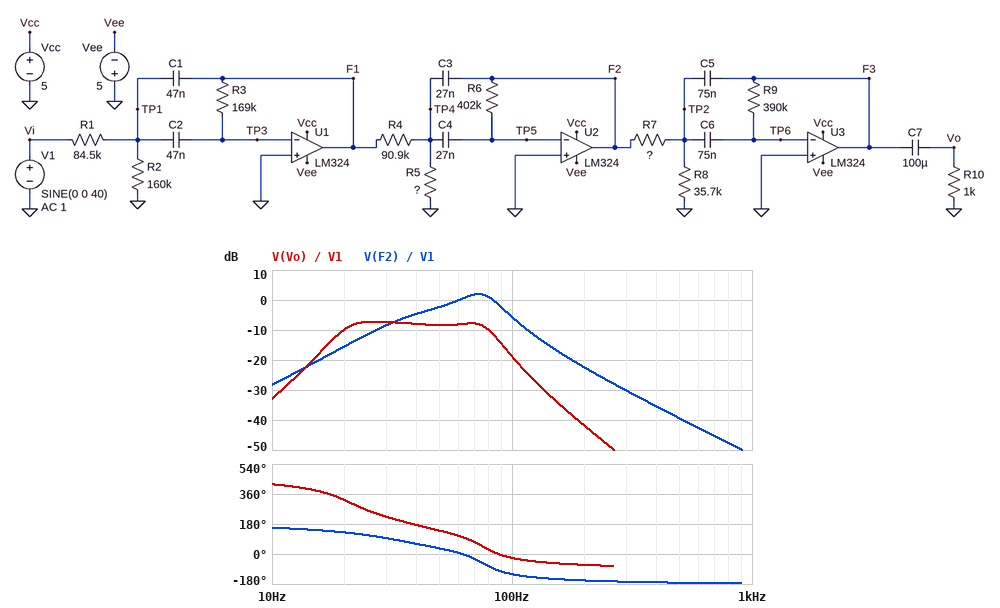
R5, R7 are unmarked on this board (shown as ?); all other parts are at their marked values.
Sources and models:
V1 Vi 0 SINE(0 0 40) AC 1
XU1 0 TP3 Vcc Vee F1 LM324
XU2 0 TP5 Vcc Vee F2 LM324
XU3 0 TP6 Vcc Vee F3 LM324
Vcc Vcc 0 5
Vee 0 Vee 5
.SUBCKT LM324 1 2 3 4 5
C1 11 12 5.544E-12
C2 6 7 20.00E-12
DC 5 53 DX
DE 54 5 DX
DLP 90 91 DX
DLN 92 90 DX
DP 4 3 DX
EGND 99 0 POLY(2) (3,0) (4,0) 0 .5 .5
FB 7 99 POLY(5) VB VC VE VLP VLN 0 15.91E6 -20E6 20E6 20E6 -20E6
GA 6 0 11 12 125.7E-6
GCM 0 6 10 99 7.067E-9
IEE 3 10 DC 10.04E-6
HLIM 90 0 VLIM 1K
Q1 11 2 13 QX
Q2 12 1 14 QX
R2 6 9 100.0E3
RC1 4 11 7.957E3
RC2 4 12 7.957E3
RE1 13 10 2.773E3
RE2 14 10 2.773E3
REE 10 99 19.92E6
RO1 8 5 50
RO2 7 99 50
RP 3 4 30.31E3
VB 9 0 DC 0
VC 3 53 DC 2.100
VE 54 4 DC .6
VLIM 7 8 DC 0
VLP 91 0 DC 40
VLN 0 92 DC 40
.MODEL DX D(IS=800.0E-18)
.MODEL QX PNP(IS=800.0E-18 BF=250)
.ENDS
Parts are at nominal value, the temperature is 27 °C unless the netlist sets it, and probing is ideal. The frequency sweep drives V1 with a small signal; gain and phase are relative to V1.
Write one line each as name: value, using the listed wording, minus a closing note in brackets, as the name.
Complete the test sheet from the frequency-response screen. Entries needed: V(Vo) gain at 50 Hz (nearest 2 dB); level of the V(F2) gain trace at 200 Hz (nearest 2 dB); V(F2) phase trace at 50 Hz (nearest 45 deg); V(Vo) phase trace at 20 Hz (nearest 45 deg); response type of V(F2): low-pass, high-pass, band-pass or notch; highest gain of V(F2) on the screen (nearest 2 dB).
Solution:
V(Vo) gain at 50 Hz: -8 dB
level of the V(F2) gain trace at 200 Hz: -22 dB
V(F2) phase trace at 50 Hz: 45 deg
V(Vo) phase trace at 20 Hz: 315 deg
response type of V(F2): low-pass, high-pass, band-pass or notch: band-pass
highest gain of V(F2) on the screen: 2 dB
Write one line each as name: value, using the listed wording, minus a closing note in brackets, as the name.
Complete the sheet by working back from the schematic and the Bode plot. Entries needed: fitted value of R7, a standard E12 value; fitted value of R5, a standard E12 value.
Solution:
fitted value of R7, a standard E12 value: 100 kΩ
fitted value of R5, a standard E12 value: 18 kΩ
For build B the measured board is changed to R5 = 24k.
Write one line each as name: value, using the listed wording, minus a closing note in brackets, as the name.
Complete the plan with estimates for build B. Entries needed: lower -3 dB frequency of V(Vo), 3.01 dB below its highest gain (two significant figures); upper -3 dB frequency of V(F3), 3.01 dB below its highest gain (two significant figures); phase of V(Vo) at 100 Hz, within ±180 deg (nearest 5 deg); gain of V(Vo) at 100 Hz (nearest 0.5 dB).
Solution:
lower -3 dB frequency of V(Vo), 3.01 dB below its highest gain: 20 Hz
upper -3 dB frequency of V(F3), 3.01 dB below its highest gain: 72 Hz
phase of V(Vo) at 100 Hz, within ±180 deg: -30 deg
gain of V(Vo) at 100 Hz: -20.5 dB
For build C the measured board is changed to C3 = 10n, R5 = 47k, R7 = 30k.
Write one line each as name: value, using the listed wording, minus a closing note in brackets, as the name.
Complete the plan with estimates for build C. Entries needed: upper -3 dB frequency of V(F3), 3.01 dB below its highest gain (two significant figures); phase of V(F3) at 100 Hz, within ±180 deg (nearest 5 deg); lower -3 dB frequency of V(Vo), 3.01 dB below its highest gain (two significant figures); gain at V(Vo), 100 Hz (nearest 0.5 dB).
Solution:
upper -3 dB frequency of V(F3), 3.01 dB below its highest gain: 41 Hz
phase of V(F3) at 100 Hz, within ±180 deg: 5 deg
lower -3 dB frequency of V(Vo), 3.01 dB below its highest gain: 24 Hz
gain at V(Vo), 100 Hz: -0.5 dB
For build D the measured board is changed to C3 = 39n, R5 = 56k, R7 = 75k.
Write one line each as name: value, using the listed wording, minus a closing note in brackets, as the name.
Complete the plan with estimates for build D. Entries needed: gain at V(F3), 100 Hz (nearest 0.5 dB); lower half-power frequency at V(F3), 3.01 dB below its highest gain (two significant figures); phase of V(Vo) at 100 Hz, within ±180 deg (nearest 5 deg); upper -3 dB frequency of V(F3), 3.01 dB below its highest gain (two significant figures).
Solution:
gain at V(F3), 100 Hz: -24.0 dB
lower half-power frequency at V(F3), 3.01 dB below its highest gain: 21 Hz
phase of V(Vo) at 100 Hz, within ±180 deg: -40 deg
upper -3 dB frequency of V(F3), 3.01 dB below its highest gain: 44 Hz
